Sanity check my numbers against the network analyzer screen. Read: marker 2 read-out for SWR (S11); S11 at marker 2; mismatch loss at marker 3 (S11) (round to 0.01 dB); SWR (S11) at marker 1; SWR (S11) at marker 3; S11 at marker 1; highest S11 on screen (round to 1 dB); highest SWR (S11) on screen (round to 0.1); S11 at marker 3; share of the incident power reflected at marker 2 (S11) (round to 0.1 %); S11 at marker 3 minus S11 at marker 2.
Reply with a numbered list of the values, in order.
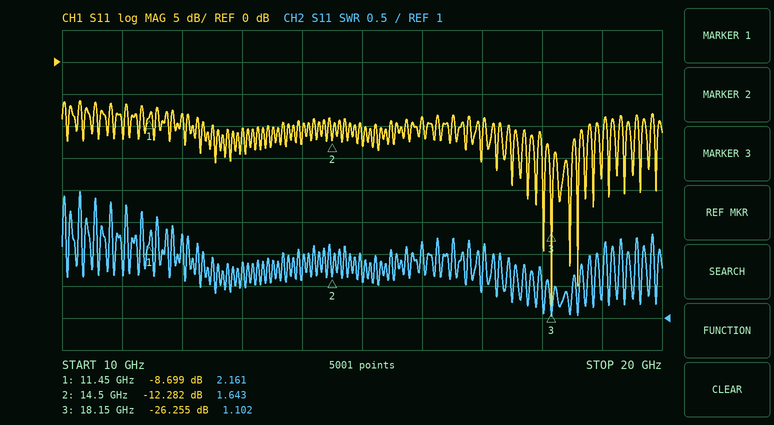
1. 1.643
2. -12.282 dB
3. 0.01 dB
4. 2.161
5. 1.102
6. -8.699 dB
7. -6 dB
8. 3.0
9. -26.255 dB
10. 5.9 %
11. -13.973 dB
